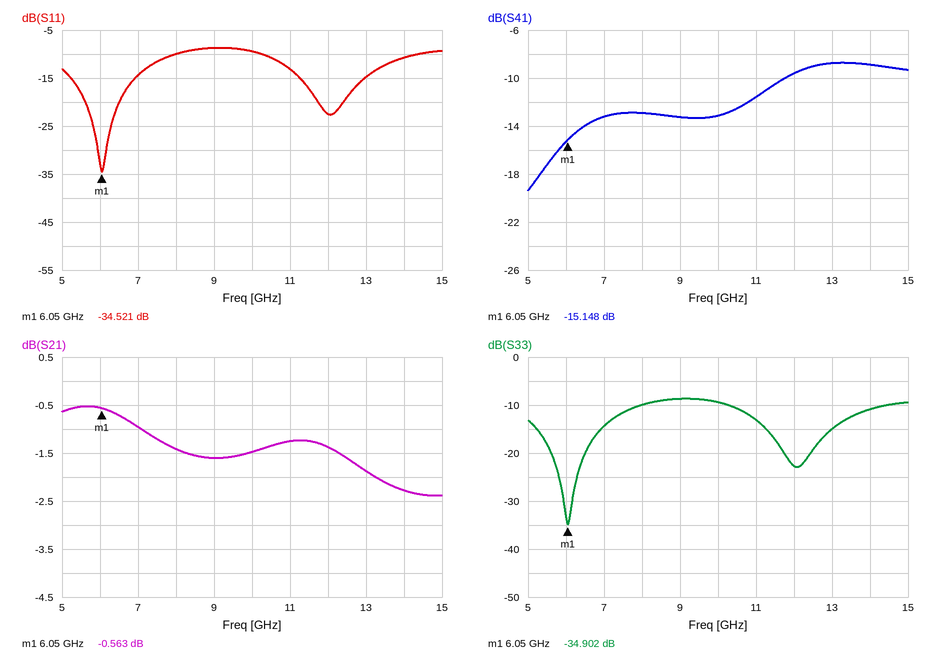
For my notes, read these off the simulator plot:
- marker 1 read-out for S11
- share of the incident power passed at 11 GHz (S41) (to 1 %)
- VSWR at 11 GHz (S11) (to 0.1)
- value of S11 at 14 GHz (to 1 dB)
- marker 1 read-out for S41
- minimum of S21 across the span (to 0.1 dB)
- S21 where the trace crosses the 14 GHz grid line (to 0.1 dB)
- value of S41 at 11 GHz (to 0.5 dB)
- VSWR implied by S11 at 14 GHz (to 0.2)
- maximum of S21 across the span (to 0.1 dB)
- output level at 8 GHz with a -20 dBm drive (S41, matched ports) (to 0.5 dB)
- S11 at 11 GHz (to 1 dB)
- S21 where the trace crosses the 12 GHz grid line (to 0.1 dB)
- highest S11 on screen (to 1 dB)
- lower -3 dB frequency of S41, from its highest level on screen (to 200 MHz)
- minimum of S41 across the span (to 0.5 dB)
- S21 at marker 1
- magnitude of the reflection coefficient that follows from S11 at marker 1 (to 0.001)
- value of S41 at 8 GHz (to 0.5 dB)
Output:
-34.521 dB
7 %
1.6
-11 dB
-15.148 dB
-2.4 dB
-2.3 dB
-11.5 dB
1.8
-0.5 dB
-33.0 dBm
-13 dB
-1.4 dB
-9 dB
11.0 GHz
-19.5 dB
-0.563 dB
0.019
-13.0 dB
